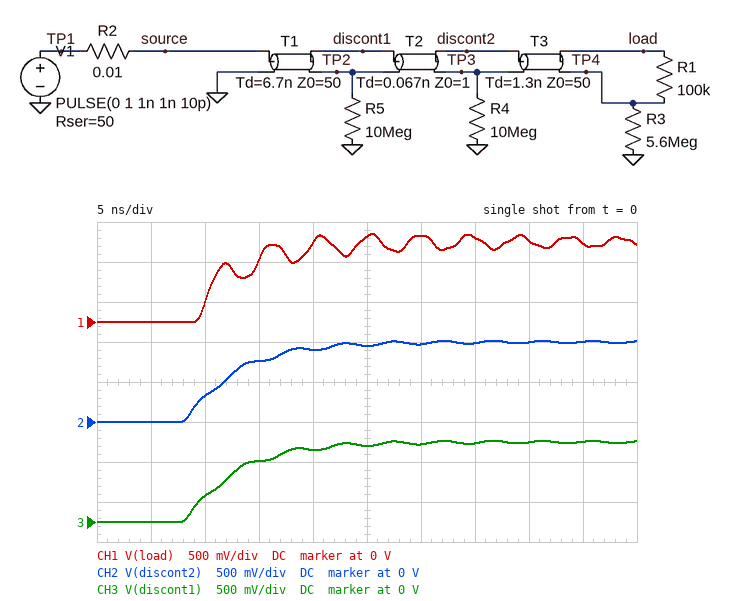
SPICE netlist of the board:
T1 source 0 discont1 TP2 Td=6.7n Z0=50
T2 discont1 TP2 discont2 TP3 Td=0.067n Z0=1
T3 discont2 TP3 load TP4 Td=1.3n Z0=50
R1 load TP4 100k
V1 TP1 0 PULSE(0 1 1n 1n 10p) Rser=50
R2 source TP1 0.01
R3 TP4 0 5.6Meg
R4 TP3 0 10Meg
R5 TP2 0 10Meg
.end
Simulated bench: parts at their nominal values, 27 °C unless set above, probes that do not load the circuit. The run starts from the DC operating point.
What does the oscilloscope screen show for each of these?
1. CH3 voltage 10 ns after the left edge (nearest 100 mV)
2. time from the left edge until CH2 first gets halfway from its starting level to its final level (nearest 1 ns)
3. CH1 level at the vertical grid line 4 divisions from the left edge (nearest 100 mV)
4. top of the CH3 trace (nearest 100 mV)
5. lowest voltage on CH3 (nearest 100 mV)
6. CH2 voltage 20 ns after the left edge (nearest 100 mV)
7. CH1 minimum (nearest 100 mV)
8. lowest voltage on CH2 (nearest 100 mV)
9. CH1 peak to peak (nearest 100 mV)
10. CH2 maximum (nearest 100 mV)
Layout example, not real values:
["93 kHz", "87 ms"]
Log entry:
["300 mV", "12 ns", "1.0 V", "1.0 V", "0 V", "900 mV", "0 V", "0 V", "1.1 V", "1.0 V"]
